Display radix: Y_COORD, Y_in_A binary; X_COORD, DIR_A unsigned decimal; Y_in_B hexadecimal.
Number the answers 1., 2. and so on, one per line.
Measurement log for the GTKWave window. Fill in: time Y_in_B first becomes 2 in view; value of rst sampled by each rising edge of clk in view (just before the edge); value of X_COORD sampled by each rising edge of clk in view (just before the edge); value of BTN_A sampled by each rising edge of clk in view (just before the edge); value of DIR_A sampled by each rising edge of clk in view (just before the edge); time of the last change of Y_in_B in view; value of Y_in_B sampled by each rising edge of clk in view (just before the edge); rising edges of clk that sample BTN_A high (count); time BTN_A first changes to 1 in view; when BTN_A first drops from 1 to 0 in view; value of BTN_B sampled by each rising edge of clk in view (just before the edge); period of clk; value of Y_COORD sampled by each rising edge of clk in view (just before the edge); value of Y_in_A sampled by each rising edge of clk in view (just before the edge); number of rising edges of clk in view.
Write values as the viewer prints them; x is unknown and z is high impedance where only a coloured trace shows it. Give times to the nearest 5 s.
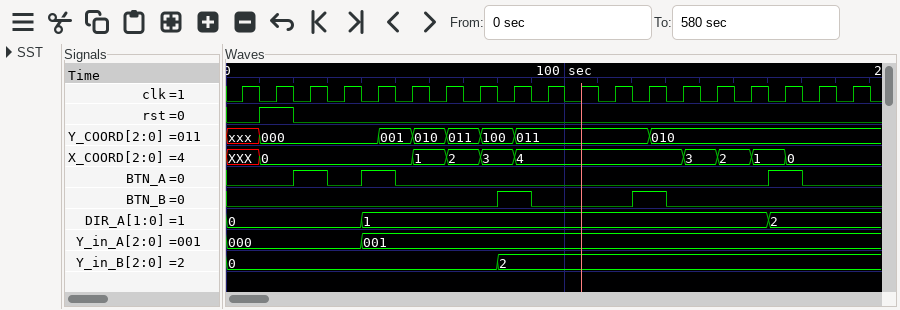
1. 80 s
2. 0 1 0 0 0 0 0 0 0 0 0 0 0 0 0 0 0 0 0
3. XXX, 0, 0, 0, 0, 0, 1, 2, 3, 4, 4, 4, 4, 4, 3, 2, 1, 0, 0
4. 0 0 1 0 1 0 0 0 0 0 0 0 0 0 0 0 1 0 0
5. 0, 0, 0, 0, 1, 1, 1, 1, 1, 1, 1, 1, 1, 1, 1, 1, 2, 2, 2
6. 80 s
7. 0, 0, 0, 0, 0, 0, 0, 0, 2, 2, 2, 2, 2, 2, 2, 2, 2, 2, 2
8. 3
9. 20 s
10. 30 s
11. 0 0 0 0 0 0 0 0 1 0 0 0 1 0 0 0 0 0 0
12. 10 s
13. xxx, 000, 000, 000, 000, 001, 010, 011, 100, 011, 011, 011, 011, 010, 010, 010, 010, 010, 010
14. 000, 000, 000, 000, 001, 001, 001, 001, 001, 001, 001, 001, 001, 001, 001, 001, 001, 001, 001
15. 19
